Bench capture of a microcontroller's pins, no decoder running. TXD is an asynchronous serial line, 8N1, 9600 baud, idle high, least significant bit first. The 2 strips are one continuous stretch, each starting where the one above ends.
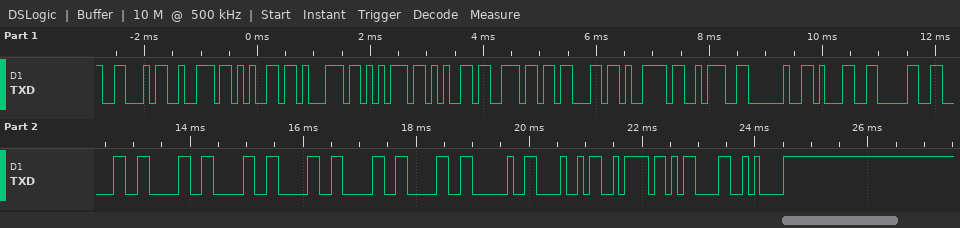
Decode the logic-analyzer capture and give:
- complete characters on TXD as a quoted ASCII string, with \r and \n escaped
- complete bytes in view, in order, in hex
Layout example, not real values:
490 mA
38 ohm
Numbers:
"Frequency: 10000000 Hz\r\n"
46 72 65 71 75 65 6E 63 79 3A 20 31 30 30 30 30 30 30 30 20 48 7A 0D 0A
